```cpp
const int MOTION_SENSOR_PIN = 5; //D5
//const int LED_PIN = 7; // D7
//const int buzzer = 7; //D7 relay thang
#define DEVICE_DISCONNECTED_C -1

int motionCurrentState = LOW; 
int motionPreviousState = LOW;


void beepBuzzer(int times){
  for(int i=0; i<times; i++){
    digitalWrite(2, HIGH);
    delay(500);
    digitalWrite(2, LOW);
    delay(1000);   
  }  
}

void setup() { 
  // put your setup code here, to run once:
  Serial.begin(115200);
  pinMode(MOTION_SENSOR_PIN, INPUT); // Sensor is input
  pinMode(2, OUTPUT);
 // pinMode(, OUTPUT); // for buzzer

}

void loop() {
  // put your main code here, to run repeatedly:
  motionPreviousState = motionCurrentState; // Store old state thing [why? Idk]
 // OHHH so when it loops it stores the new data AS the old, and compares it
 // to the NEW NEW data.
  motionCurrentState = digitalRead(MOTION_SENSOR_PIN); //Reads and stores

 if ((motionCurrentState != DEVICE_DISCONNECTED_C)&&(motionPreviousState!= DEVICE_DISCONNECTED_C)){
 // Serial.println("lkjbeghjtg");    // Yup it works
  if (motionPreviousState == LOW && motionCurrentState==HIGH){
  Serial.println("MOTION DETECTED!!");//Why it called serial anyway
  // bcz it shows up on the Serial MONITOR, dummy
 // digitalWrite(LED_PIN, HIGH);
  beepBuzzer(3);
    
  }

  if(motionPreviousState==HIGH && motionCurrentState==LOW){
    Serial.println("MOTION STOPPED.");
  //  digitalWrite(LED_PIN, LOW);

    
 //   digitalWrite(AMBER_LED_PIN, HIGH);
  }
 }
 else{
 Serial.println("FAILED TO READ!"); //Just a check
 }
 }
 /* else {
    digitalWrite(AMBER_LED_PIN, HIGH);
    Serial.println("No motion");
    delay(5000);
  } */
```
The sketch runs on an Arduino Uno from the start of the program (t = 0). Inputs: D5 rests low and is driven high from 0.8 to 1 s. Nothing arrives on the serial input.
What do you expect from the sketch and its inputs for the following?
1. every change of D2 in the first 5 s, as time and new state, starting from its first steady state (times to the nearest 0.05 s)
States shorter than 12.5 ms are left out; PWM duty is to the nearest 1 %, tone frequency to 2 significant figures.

0 s low; 0.8 s high; 1.3 s low; 2.3 s high; 2.8 s low; 3.8 s high; 4.3 s low
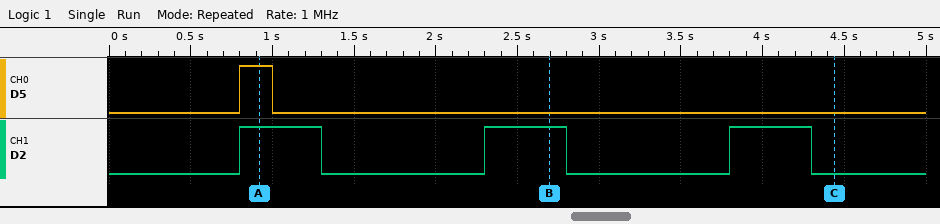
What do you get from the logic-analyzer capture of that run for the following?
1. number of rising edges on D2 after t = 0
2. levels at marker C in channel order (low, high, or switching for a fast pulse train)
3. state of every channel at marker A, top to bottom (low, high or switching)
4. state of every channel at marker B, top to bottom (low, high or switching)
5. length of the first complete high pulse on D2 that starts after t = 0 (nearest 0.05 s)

3
D5 low, D2 low
D5 high, D2 high
D5 low, D2 high
0.50 s
